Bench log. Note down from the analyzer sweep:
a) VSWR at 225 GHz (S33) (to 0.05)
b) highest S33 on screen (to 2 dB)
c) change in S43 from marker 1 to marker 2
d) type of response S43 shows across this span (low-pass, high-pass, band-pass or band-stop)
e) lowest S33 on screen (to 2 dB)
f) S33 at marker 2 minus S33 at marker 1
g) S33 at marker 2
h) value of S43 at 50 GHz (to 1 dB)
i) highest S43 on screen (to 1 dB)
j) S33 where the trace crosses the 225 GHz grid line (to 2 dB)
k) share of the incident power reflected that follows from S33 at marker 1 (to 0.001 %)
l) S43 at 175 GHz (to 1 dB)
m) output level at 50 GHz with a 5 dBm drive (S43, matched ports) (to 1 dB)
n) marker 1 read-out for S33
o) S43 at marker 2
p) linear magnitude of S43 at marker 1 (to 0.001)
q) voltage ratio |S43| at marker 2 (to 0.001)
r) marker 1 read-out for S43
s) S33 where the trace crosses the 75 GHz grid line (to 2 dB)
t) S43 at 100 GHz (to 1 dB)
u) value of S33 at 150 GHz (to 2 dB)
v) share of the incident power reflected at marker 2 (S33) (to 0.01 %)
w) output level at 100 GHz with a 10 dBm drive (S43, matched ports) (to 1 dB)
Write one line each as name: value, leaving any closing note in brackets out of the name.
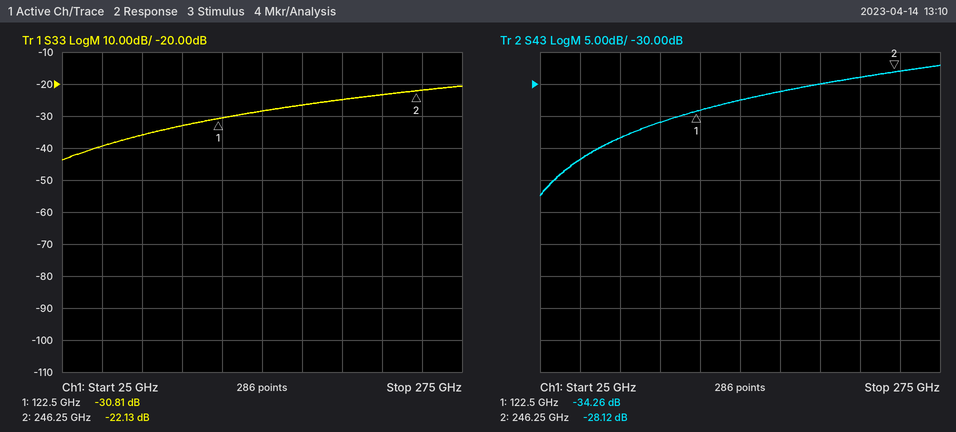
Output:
VSWR at 225 GHz (S33): 1.15
highest S33 on screen: -20 dB
change in S43 from marker 1 to marker 2: 6.14 dB
type of response S43 shows across this span: high-pass
lowest S33 on screen: -44 dB
S33 at marker 2 minus S33 at marker 1: 8.68 dB
S33 at marker 2: -22.13 dB
value of S43 at 50 GHz: -42 dB
highest S43 on screen: -27 dB
S33 where the trace crosses the 225 GHz grid line: -24 dB
share of the incident power reflected that follows from S33 at marker 1: 0.083 %
S43 at 175 GHz: -31 dB
output level at 50 GHz with a 5 dBm drive (S43, matched ports): -37 dBm
marker 1 read-out for S33: -30.81 dB
S43 at marker 2: -28.12 dB
linear magnitude of S43 at marker 1: 0.019
voltage ratio |S43| at marker 2: 0.039
marker 1 read-out for S43: -34.26 dB
S33 where the trace crosses the 75 GHz grid line: -36 dB
S43 at 100 GHz: -36 dB
value of S33 at 150 GHz: -28 dB
share of the incident power reflected at marker 2 (S33): 0.61 %
output level at 100 GHz with a 10 dBm drive (S43, matched ports): -26 dBm
